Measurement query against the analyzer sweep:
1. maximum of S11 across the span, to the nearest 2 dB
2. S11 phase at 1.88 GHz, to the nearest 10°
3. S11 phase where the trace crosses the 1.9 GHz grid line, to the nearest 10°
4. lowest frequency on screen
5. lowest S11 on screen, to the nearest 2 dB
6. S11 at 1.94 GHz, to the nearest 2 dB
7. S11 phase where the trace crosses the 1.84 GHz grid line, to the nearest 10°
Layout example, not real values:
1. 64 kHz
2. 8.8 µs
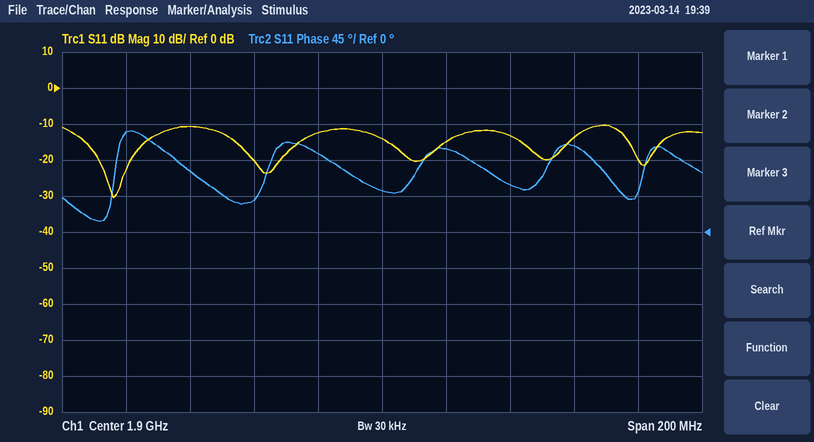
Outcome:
1. -10 dB
2. 100°
3. 50°
4. 1.8 GHz
5. -30 dB
6. -14 dB
7. 80°
